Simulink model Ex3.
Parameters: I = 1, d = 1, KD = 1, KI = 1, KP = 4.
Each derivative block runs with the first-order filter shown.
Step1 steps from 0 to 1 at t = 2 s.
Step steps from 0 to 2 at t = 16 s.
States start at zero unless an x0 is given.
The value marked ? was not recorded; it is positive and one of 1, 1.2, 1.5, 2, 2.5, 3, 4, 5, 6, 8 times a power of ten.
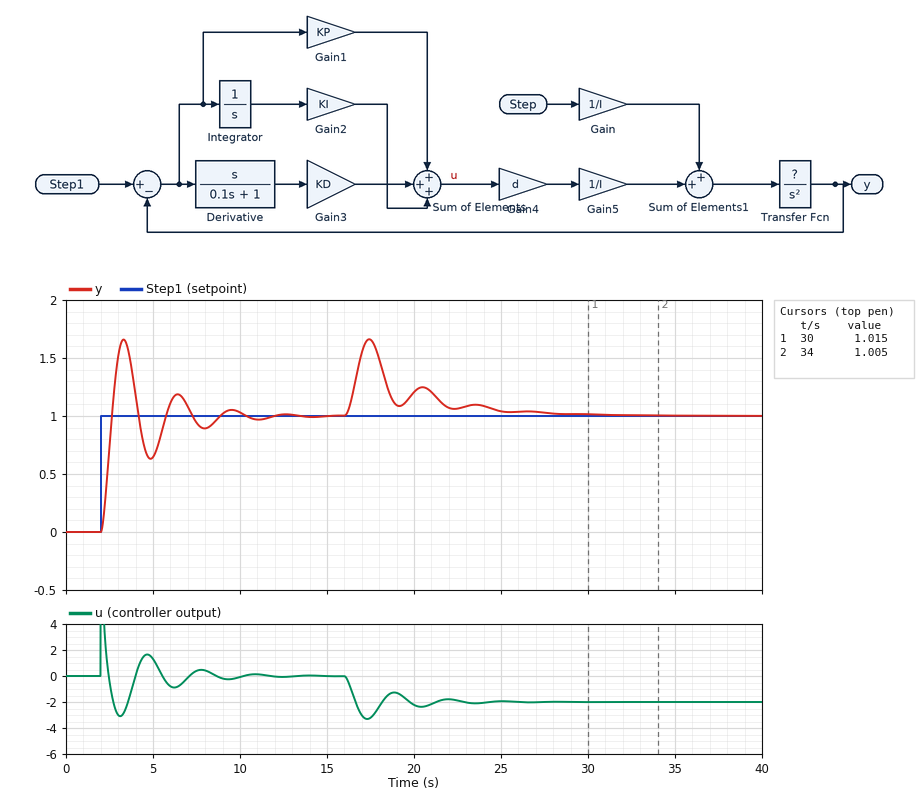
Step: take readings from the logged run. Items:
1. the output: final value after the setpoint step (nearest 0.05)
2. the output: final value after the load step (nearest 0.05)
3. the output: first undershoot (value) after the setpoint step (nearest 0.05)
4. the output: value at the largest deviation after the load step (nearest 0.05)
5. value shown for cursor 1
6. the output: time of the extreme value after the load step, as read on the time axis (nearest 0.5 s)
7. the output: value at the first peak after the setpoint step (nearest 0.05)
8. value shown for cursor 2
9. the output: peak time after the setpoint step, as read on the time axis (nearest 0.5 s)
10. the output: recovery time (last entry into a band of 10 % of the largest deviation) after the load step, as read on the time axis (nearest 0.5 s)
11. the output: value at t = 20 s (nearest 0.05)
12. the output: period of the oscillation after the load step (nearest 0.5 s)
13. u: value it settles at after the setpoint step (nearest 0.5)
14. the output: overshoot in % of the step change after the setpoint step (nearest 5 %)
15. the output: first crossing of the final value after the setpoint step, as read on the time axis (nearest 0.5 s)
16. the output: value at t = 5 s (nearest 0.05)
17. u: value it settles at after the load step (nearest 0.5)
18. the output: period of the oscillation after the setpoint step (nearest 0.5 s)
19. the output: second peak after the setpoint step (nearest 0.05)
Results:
1.00
1.00
0.65
1.65
1.015
17.5 s
1.65
1.005
3.5 s
24.5 s
1.20
3.0 s
0.0
65 %
2.5 s
0.65
-2.0
3.0 s
1.20
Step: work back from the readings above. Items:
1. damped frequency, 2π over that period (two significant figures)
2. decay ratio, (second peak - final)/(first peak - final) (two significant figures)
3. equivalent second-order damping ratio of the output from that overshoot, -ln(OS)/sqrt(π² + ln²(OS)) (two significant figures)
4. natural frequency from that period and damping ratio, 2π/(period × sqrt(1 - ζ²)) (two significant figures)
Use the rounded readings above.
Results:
2.1 rad/s
0.31
0.14
2.1 rad/s
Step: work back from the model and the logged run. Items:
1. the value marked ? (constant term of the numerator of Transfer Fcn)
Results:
1
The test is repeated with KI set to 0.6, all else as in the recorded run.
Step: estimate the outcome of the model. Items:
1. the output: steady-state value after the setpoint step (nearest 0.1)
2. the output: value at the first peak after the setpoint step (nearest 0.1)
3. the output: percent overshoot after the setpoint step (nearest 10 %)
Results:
1.0
1.6
60 %
